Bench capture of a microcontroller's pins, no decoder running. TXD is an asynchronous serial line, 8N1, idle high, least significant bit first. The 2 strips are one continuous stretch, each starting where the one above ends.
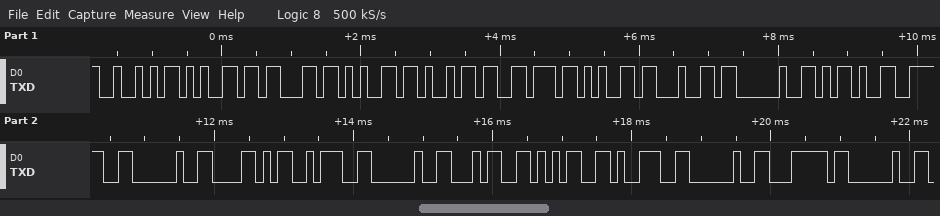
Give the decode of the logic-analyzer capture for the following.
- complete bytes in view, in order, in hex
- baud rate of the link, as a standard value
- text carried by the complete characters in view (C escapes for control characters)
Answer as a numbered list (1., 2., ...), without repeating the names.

1. 52 65 63 65 69 76 65 64 20 2D 3E 20 58 3A 20 34 35 39 20 7C 20
2. 9600 baud
3. "Received -> X: 459 | "
